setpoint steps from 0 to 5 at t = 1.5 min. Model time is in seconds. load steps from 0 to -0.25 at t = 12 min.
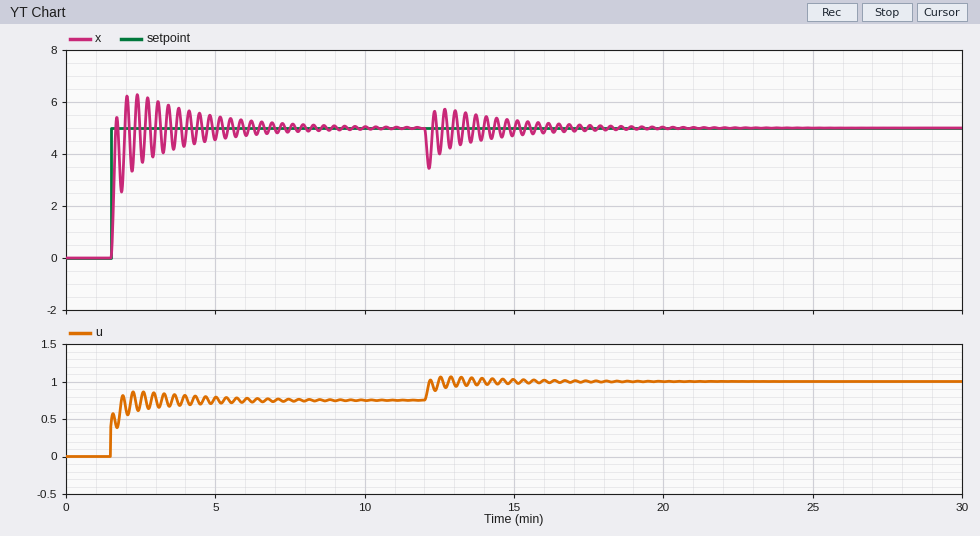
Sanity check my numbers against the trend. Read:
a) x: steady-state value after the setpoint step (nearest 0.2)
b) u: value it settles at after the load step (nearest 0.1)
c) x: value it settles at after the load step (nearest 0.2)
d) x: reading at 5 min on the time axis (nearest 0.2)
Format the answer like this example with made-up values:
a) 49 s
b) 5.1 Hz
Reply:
a) 5.0
b) 1.0
c) 5.0
d) 4.6
